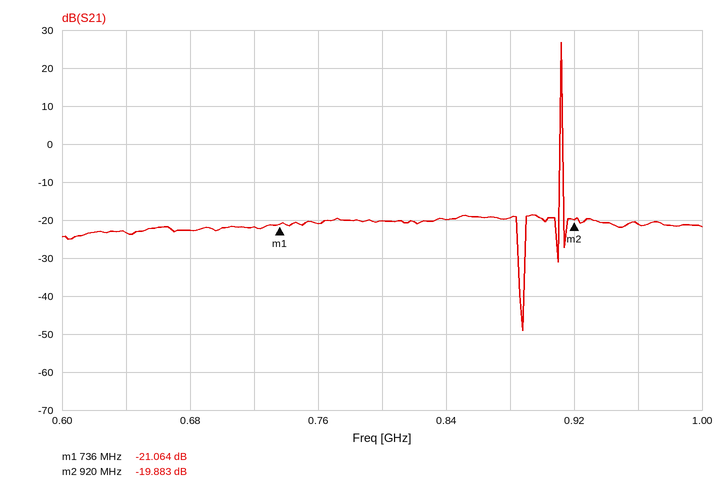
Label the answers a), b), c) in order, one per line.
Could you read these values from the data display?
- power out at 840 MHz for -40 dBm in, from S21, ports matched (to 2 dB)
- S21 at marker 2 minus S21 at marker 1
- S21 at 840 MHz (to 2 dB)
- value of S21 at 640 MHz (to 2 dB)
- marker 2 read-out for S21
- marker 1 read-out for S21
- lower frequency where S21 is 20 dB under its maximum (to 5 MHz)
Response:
a) -60 dBm
b) 1.181 dB
c) -20 dB
d) -24 dB
e) -19.883 dB
f) -21.064 dB
g) 910 MHz
